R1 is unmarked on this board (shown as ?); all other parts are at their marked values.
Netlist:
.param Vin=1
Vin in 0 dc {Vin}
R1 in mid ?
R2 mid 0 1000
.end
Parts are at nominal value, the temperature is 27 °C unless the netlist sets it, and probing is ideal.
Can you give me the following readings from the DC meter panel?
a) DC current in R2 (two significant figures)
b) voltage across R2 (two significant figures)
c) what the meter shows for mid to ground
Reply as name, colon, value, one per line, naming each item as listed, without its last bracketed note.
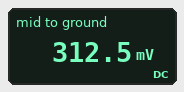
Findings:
DC current in R2: 310 µA
voltage across R2: 310 mV
what the meter shows for mid to ground: 312.5 mV
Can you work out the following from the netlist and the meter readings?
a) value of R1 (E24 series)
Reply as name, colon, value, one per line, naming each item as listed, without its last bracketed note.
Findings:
value of R1: 2.2 kΩ
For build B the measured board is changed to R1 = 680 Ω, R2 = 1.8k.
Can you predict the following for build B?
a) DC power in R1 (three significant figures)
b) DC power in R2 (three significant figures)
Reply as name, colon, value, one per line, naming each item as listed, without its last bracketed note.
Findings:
DC power in R1: 111 µW
DC power in R2: 293 µW
